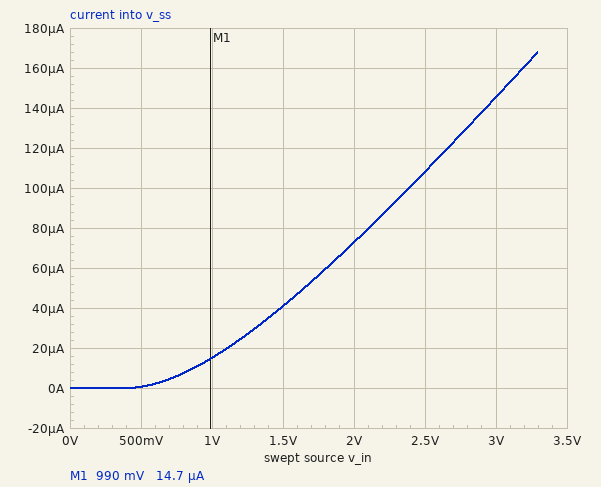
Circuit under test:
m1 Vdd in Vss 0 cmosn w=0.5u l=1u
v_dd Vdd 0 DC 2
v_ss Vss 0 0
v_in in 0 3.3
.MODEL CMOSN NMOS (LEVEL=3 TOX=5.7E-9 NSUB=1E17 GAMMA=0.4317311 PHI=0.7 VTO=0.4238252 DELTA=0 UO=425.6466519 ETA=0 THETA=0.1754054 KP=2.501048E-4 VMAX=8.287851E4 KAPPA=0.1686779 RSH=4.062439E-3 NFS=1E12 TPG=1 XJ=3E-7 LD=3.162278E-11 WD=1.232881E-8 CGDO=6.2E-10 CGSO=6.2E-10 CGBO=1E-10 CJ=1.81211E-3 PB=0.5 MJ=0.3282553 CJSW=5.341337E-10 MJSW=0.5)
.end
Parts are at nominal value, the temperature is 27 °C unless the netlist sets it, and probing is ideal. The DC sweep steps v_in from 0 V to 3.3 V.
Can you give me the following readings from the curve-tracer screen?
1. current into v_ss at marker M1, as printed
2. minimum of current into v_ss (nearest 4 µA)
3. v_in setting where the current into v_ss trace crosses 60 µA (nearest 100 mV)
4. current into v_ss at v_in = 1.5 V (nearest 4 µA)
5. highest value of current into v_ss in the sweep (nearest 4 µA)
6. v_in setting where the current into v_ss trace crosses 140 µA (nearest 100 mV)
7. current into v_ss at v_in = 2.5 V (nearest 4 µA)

14.7 µA
0 A
1.8 V
40 µA
168 µA
2.9 V
108 µA
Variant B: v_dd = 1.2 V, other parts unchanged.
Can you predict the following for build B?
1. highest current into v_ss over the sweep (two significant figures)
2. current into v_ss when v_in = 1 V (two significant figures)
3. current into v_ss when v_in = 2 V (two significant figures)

150 µA
15 µA
71 µA
